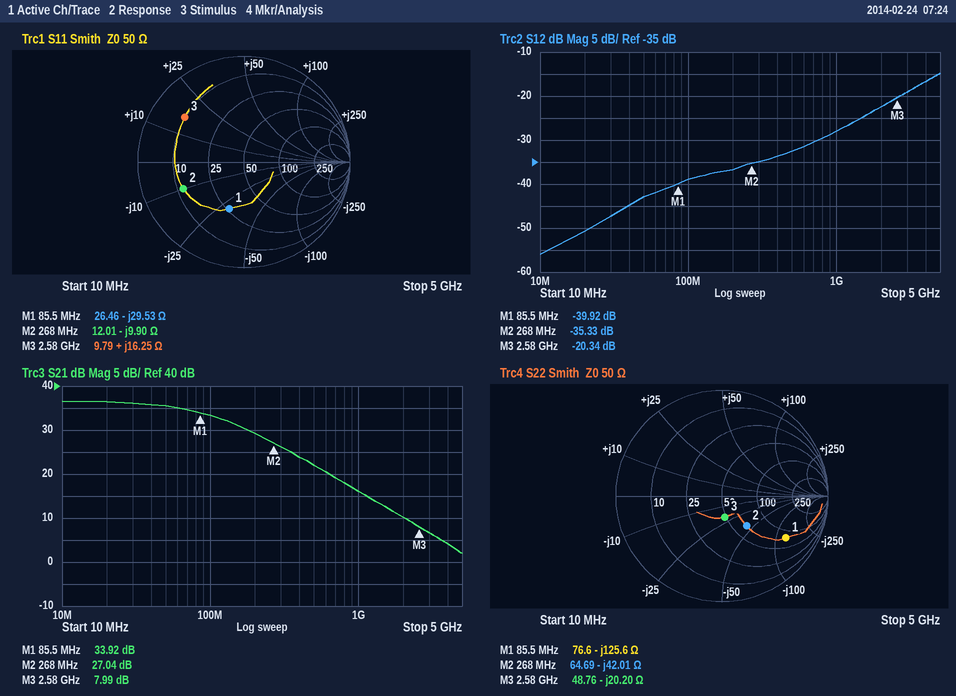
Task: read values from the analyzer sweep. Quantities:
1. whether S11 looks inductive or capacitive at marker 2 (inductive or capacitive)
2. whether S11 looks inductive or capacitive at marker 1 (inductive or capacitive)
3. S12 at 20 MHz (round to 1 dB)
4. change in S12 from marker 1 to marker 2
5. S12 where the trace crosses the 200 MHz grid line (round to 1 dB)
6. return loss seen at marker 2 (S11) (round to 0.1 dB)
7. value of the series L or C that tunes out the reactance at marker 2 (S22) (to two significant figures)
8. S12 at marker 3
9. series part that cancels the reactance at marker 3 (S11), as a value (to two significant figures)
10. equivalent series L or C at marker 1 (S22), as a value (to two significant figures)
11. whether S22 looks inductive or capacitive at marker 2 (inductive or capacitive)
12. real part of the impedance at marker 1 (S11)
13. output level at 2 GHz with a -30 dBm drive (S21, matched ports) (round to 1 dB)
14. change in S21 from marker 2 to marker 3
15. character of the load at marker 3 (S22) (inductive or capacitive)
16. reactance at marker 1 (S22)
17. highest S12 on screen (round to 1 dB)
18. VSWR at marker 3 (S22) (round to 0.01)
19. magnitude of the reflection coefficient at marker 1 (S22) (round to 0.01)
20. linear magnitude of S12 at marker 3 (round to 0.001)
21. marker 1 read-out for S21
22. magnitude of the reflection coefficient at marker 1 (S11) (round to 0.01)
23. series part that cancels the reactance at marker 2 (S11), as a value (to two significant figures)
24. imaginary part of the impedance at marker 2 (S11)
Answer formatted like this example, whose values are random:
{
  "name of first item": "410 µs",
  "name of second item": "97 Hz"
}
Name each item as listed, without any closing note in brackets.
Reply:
{
  "whether S11 looks inductive or capacitive at marker 2": "capacitive",
  "whether S11 looks inductive or capacitive at marker 1": "capacitive",
  "S12 at 20 MHz": "-51 dB",
  "change in S12 from marker 1 to marker 2": "4.59 dB",
  "S12 where the trace crosses the 200 MHz grid line": "-37 dB",
  "return loss seen at marker 2 (S11)": "4.1 dB",
  "value of the series L or C that tunes out the reactance at marker 2 (S22)": "25 nH",
  "S12 at marker 3": "-20.34 dB",
  "series part that cancels the reactance at marker 3 (S11), as a value": "3.8 pF",
  "equivalent series L or C at marker 1 (S22), as a value": "15 pF",
  "whether S22 looks inductive or capacitive at marker 2": "capacitive",
  "real part of the impedance at marker 1": "26.46 Ω",
  "output level at 2 GHz with a -30 dBm drive (S21, matched ports)": "-20 dBm",
  "change in S21 from marker 2 to marker 3": "-19.05 dB",
  "character of the load at marker 3 (S22)": "capacitive",
  "reactance at marker 1": "-125.6 Ω",
  "highest S12 on screen": "-15 dB",
  "VSWR at marker 3 (S22)": "1.50",
  "magnitude of the reflection coefficient at marker 1 (S22)": "0.72",
  "linear magnitude of S12 at marker 3": "0.096",
  "marker 1 read-out for S21": "33.92 dB",
  "magnitude of the reflection coefficient at marker 1 (S11)": "0.46",
  "series part that cancels the reactance at marker 2 (S11), as a value": "5.9 nH",
  "imaginary part of the impedance at marker 2": "-9.90 Ω"
}
